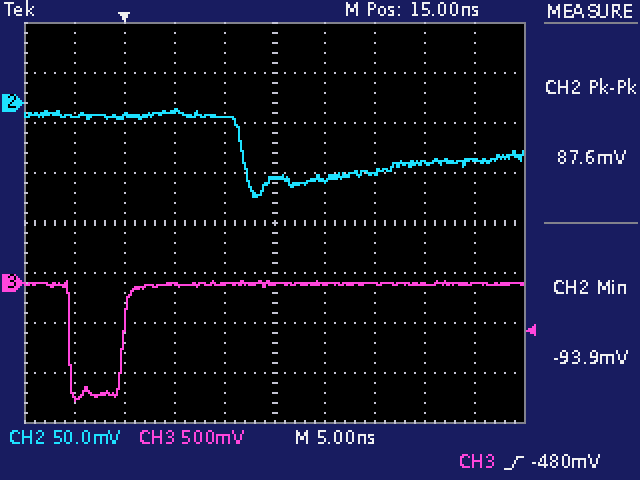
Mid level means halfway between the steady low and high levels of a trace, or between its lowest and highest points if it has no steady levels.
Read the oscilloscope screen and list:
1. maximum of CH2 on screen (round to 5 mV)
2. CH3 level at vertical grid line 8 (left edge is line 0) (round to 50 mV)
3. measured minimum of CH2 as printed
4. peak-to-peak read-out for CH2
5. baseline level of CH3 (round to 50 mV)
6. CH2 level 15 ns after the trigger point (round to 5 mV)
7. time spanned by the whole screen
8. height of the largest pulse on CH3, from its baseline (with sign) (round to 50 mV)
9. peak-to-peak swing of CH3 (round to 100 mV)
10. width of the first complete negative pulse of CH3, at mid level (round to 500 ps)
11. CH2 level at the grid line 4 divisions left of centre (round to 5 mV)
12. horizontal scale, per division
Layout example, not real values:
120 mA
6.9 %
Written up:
-5 mV
0 mV
-93.9 mV
87.6 mV
0 mV
-75 mV
50 ns
-1.15 V
1.20 V
5.5 ns
-15 mV
5 ns
